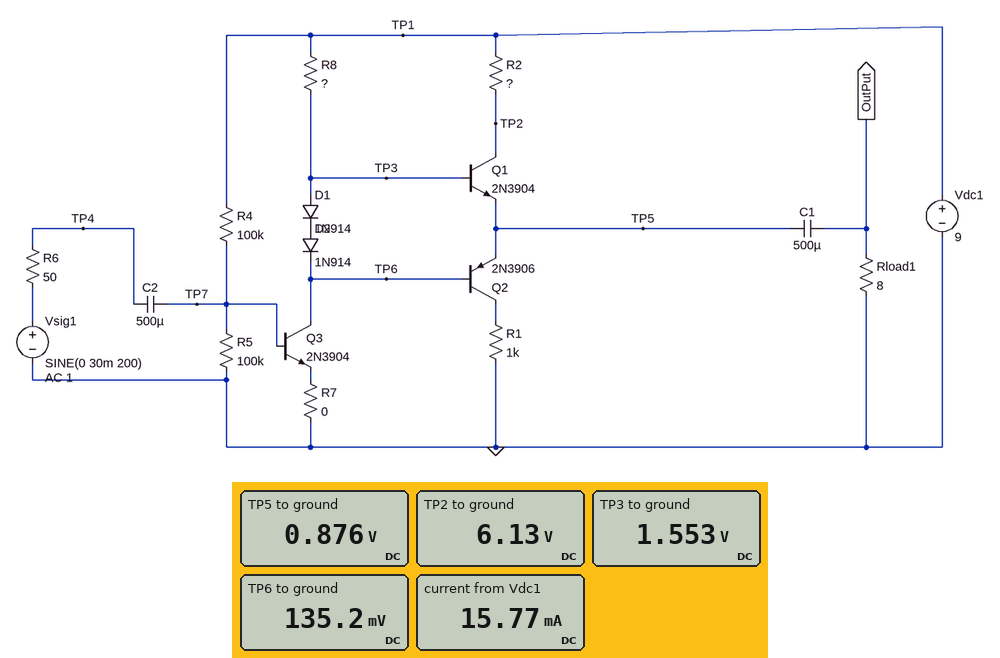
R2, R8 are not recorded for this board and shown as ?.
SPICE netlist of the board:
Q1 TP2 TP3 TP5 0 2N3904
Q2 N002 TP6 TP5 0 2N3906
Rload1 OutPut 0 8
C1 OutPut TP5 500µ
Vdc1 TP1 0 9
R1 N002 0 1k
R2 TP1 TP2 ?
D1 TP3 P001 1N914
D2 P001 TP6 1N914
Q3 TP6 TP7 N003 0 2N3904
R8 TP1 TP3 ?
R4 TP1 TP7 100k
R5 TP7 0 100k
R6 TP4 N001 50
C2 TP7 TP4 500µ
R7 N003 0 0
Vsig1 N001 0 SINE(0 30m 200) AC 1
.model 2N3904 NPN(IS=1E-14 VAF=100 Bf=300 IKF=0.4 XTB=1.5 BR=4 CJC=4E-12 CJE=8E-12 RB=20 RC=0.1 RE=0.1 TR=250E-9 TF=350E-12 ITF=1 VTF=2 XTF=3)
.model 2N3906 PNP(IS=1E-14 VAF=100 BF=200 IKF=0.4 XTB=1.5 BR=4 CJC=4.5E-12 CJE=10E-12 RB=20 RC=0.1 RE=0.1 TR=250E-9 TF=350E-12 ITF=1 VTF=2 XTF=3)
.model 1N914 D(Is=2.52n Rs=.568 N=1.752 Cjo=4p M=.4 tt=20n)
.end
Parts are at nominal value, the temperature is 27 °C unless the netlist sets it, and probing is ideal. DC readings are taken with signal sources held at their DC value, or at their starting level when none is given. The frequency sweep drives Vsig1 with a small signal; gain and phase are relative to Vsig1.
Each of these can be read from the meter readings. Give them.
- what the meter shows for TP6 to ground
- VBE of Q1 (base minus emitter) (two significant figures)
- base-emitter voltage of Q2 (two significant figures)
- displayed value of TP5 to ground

135.2 mV
680 mV
-740 mV
0.876 V
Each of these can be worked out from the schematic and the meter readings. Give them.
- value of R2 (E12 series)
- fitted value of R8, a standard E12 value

1.2 kΩ
560 Ω
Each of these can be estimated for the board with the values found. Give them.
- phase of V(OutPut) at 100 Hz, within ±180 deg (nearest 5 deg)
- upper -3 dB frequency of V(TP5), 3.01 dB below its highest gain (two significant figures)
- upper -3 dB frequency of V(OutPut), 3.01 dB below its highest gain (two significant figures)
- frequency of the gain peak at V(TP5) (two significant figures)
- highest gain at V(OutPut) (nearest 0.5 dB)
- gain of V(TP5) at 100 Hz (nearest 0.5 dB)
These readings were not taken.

-170 deg
23 Hz
240 kHz
7.5 Hz
12.5 dB
13.0 dB
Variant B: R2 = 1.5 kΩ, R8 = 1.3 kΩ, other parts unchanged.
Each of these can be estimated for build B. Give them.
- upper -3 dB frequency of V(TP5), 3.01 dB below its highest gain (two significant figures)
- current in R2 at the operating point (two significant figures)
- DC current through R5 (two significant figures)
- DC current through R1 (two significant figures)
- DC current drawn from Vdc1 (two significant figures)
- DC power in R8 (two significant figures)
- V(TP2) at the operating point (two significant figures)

16 Hz
1.0 mA
7.1 µA
750 µA
6.9 mA
44 mW
7.5 V
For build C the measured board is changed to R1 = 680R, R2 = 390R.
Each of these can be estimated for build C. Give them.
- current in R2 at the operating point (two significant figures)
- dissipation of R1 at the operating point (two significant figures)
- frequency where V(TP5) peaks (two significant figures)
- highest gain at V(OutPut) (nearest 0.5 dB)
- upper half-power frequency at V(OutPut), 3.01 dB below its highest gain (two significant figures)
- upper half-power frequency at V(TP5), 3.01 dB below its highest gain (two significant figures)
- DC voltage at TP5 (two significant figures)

2.7 mA
1.1 mW
7.8 Hz
13.0 dB
230 kHz
25 Hz
870 mV
